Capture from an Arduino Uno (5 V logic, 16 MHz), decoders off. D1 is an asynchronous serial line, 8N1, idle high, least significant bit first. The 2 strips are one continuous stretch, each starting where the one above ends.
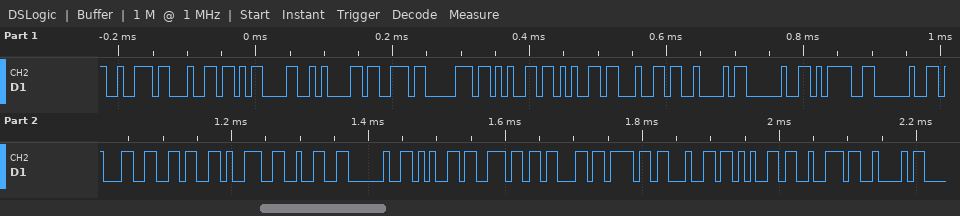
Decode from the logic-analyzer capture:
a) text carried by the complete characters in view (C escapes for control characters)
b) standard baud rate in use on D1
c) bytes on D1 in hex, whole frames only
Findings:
"rd\r\nspeedB = 1692 encoderB"
115200 baud
0x72 0x64 0x0D 0x0A 0x73 0x70 0x65 0x65 0x64 0x42 0x20 0x3D 0x20 0x31 0x36 0x39 0x32 0x20 0x65 0x6E 0x63 0x6F 0x64 0x65 0x72 0x42
